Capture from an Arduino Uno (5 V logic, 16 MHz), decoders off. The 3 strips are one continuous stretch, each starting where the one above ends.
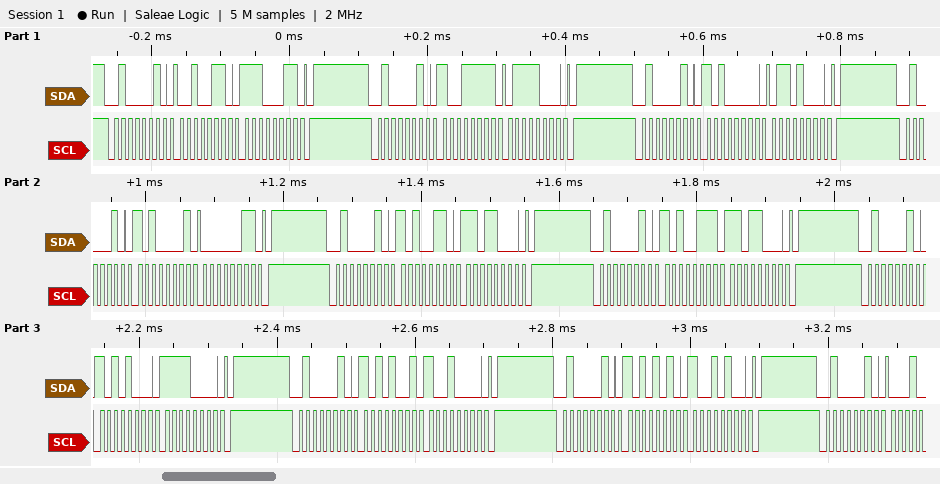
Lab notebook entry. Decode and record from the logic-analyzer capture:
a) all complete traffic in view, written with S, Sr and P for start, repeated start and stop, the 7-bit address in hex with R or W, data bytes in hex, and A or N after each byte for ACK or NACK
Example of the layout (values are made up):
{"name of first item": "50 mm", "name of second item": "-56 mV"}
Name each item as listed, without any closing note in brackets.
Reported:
{"all complete traffic in view, written with S, Sr and P for start, repeated start and stop, the 7-bit address in hex with R or W, data bytes in hex, and A or N after each byte for ACK or NACK": "S 21W A 26 A E3 A P S 21W A 9F A 78 A P S 21W A A0 A 68 A P S 21W A A1 A 03 A P S 21W A A6 A D8 A P S 21W A A7 A D8 A P S 21W A A8 A F0 A P S 21W A A9 A 90 A P S 21W A AA A 94 A P S 21W A"}
